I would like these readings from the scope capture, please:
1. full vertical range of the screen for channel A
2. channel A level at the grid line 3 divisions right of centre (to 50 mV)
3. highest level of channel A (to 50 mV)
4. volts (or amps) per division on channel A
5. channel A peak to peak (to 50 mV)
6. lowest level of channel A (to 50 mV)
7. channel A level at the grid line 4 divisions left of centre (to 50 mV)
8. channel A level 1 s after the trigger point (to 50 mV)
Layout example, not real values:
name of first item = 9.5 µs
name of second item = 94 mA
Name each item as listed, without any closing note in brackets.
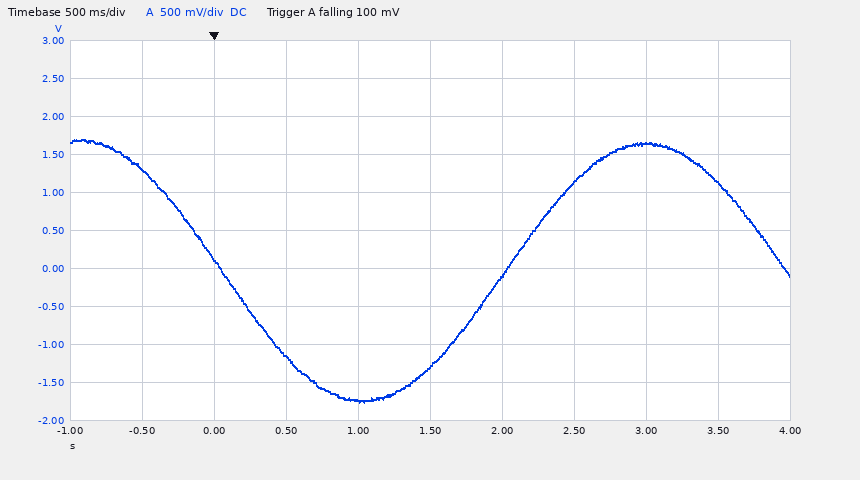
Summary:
full vertical range of the screen for channel A = 5 V
channel A level at the grid line 3 divisions right of centre = 1.65 V
highest level of channel A = 1.70 V
volts (or amps) per division on channel A = 500 mV
channel A peak to peak = 3.45 V
lowest level of channel A = -1.75 V
channel A level at the grid line 4 divisions left of centre = 1.30 V
channel A level 1 s after the trigger point = -1.75 V
